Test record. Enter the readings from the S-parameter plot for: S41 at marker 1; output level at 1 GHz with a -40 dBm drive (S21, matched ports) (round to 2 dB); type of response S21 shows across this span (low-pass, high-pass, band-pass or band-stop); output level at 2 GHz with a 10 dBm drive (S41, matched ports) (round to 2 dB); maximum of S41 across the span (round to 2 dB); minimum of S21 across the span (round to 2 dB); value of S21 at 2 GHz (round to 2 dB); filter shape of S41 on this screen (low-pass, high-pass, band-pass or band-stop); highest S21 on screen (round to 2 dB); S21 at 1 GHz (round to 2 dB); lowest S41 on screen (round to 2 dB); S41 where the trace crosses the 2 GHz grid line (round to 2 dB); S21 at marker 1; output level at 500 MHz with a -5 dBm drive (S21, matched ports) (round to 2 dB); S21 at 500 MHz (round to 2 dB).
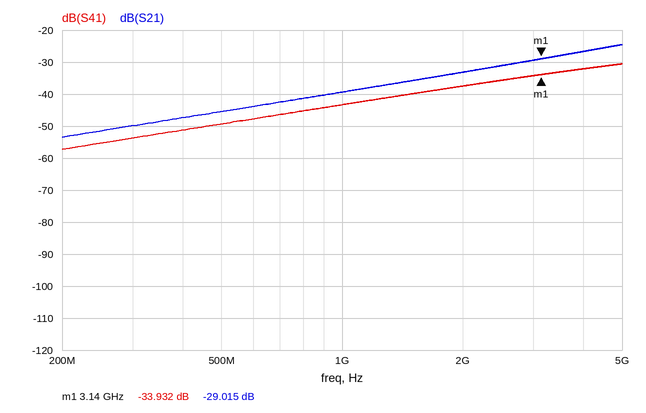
-33.932 dB
-80 dBm
high-pass
-28 dBm
-30 dB
-54 dB
-34 dB
high-pass
-24 dB
-40 dB
-58 dB
-38 dB
-29.015 dB
-50 dBm
-46 dB
